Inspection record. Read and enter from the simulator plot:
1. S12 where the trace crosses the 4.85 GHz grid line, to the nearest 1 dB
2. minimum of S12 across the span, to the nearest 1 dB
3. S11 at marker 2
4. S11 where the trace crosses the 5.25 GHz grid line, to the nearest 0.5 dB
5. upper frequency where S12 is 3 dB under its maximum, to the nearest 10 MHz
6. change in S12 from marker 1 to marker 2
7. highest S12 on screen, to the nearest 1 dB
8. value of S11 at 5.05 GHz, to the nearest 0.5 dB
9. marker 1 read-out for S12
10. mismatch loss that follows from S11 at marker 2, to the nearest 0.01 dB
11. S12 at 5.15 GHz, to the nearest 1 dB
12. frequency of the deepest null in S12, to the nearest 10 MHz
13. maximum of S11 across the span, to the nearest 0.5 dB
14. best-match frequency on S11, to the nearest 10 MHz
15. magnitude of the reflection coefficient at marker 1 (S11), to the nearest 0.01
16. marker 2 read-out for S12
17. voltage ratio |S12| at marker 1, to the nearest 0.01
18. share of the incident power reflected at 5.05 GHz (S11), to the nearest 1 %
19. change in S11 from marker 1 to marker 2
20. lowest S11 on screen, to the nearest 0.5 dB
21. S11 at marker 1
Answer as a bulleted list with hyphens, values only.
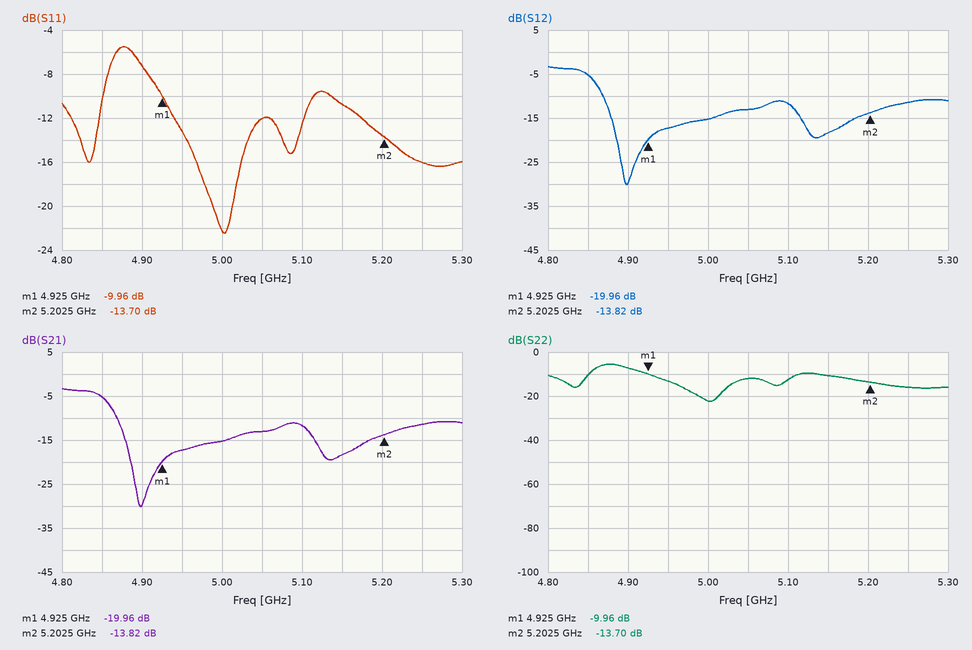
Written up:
- -5 dB
- -30 dB
- -13.70 dB
- -16.0 dB
- 4.86 GHz
- 6.14 dB
- -3 dB
- -12.0 dB
- -19.96 dB
- 0.19 dB
- -18 dB
- 4.90 GHz
- -5.5 dB
- 5.00 GHz
- 0.32
- -13.82 dB
- 0.10
- 6 %
- -3.74 dB
- -22.5 dB
- -9.96 dB
